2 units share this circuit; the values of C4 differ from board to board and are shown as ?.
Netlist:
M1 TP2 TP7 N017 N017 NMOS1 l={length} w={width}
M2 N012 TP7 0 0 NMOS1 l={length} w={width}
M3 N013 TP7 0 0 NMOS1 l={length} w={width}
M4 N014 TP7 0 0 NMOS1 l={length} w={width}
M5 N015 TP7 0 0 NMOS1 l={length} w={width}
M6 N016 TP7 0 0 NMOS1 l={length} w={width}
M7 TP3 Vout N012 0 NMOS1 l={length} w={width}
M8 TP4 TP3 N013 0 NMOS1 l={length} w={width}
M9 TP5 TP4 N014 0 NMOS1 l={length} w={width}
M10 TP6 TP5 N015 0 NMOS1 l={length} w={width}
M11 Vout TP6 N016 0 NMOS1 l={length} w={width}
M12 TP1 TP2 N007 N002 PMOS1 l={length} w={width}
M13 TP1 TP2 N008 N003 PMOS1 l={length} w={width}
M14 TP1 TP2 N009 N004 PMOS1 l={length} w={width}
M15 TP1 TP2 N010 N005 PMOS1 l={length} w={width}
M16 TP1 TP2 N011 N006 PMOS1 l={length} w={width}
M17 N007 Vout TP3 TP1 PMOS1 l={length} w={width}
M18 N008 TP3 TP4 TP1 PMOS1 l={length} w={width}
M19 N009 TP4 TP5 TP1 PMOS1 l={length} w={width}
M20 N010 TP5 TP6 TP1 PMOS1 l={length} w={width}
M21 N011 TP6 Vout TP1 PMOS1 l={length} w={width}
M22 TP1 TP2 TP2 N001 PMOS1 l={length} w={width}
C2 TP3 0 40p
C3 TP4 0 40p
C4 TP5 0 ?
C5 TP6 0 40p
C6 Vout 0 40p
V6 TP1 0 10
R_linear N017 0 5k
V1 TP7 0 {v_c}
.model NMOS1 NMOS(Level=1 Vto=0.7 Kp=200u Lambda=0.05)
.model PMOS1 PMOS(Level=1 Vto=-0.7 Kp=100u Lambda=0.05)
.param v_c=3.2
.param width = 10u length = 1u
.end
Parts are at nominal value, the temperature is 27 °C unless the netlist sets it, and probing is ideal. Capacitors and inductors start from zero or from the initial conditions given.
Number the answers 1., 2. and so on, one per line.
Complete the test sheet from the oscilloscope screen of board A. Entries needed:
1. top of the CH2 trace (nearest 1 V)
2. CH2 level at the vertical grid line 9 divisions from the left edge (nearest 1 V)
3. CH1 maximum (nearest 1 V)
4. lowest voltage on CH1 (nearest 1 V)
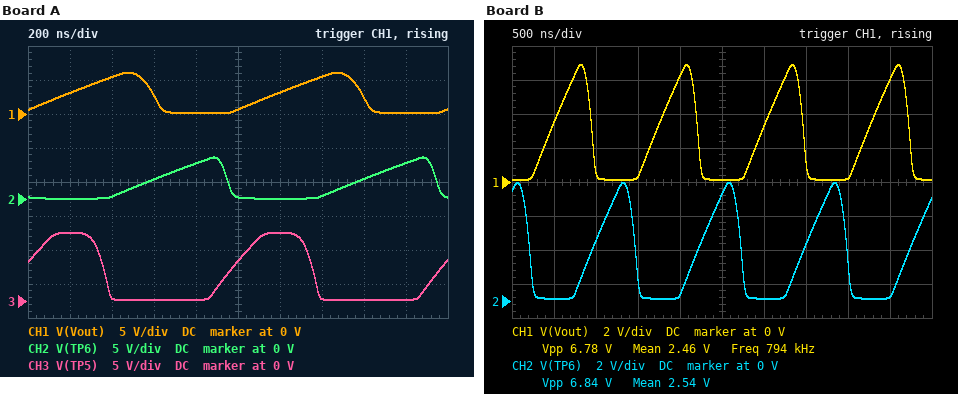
1. 6 V
2. 5 V
3. 6 V
4. 0 V
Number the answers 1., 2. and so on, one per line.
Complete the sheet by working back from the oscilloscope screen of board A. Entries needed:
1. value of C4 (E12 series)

1. 12 pF
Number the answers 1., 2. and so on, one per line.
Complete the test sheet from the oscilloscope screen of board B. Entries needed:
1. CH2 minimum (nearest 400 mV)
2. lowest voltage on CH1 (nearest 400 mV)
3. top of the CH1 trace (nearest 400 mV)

1. 0 V
2. 0 V
3. 6.8 V
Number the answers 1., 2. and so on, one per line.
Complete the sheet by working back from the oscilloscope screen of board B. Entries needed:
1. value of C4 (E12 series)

1. 47 pF
